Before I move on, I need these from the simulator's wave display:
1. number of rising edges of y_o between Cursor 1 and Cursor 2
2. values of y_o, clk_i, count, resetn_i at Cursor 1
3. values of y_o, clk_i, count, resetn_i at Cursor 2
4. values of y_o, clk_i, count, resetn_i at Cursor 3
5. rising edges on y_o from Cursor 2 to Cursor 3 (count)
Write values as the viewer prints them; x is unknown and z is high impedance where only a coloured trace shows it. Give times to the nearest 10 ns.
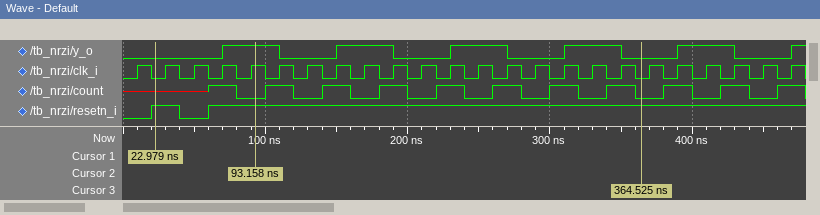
1
y_o=0, clk_i=0, count=x, resetn_i=1
y_o=1, clk_i=1, count=0, resetn_i=1
y_o=0, clk_i=0, count=0, resetn_i=1
3
